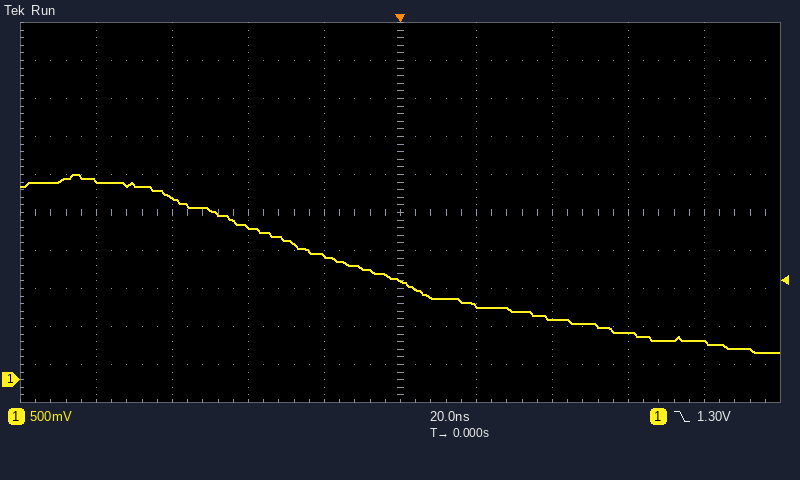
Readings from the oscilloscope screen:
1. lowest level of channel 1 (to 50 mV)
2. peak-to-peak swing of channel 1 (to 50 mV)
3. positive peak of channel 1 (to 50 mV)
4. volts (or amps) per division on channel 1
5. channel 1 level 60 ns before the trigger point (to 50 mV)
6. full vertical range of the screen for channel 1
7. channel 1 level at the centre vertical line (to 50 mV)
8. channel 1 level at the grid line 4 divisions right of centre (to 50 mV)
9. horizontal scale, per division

350 mV
2.35 V
2.70 V
500 mV
2.40 V
5 V
1.30 V
500 mV
20 ns
